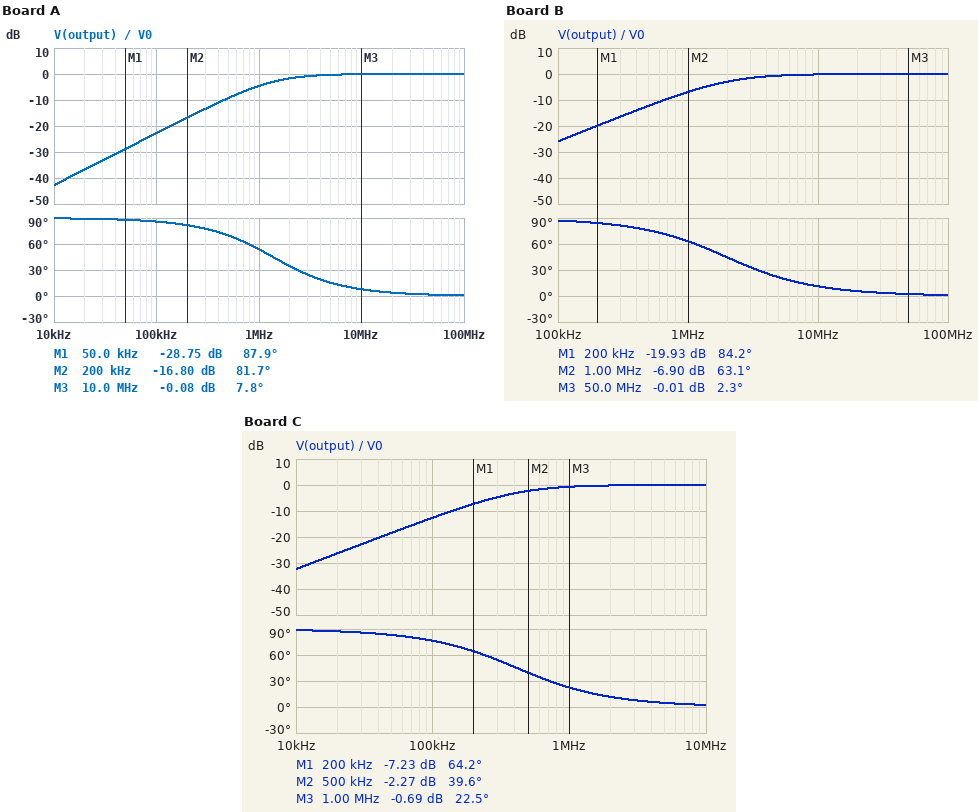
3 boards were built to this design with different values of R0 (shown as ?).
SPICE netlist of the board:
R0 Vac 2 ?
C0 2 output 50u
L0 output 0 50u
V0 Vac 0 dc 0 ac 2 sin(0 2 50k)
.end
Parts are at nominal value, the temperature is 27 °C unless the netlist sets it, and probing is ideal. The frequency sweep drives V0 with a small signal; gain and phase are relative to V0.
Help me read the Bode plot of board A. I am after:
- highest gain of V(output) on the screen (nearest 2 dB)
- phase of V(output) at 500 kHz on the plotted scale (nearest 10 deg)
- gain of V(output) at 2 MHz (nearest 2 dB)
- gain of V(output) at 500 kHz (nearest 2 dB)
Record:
0 dB
70 deg
-2 dB
-10 dB
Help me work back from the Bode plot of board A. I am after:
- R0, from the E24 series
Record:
430 Ω
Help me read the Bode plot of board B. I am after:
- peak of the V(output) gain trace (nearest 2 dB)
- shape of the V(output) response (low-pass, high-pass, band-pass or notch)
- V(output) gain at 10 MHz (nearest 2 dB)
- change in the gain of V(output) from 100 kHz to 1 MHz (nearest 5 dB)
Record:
0 dB
high-pass
0 dB
20 dB
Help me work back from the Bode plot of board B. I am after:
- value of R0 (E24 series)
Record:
620 Ω
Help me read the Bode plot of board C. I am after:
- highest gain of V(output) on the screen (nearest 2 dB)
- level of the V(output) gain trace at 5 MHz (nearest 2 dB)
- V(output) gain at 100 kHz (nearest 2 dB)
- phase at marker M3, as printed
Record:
0 dB
0 dB
-12 dB
22.5 deg
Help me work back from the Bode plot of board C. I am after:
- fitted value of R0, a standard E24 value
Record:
130 Ω
